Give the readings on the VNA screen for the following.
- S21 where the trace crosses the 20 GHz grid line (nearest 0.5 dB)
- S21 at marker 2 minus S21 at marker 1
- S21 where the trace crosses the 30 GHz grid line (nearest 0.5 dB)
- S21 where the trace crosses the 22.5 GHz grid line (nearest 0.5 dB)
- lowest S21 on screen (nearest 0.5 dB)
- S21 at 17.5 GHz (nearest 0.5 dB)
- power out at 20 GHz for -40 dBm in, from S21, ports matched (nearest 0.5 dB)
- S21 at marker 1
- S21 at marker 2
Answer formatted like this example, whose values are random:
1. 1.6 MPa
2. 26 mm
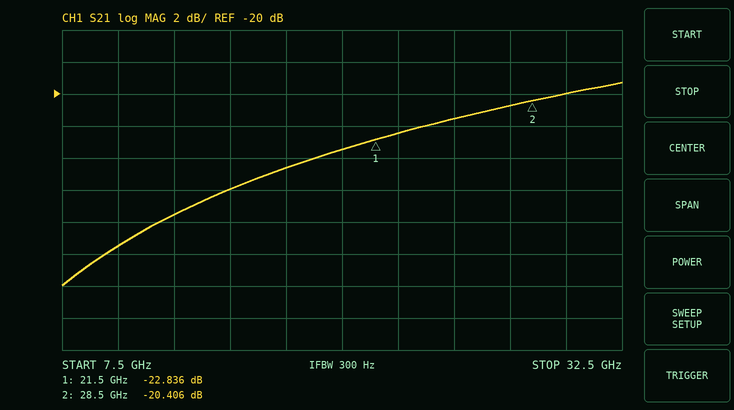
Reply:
1. -23.5 dB
2. 2.430 dB
3. -20.0 dB
4. -22.5 dB
5. -32.0 dB
6. -24.5 dB
7. -63.5 dBm
8. -22.836 dB
9. -20.406 dB
